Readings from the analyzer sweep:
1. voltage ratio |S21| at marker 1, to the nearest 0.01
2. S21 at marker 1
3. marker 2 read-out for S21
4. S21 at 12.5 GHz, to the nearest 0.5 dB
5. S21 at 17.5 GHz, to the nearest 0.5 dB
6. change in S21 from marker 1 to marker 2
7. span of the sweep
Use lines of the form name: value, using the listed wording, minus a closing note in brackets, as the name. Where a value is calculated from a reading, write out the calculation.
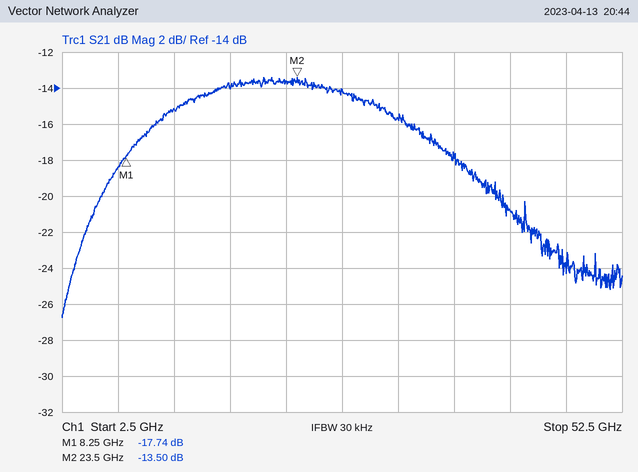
voltage ratio |S21| at marker 1, to the nearest 0.01: 10^(-17.74/20) ≈ 0.13
S21 at marker 1: -17.74 dB
marker 2 read-out for S21: -13.50 dB
S21 at 12.5 GHz, to the nearest 0.5 dB: -15.0 dB
S21 at 17.5 GHz, to the nearest 0.5 dB: -14.0 dB
change in S21 from marker 1 to marker 2: -13.5 − (-17.74) = 4.24 dB
span of the sweep: 50 GHz
